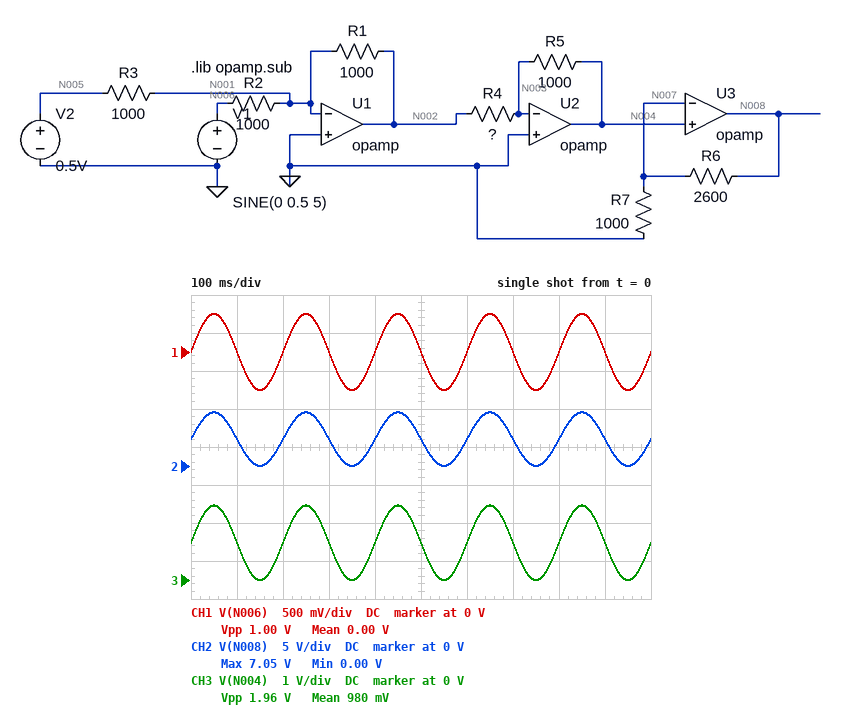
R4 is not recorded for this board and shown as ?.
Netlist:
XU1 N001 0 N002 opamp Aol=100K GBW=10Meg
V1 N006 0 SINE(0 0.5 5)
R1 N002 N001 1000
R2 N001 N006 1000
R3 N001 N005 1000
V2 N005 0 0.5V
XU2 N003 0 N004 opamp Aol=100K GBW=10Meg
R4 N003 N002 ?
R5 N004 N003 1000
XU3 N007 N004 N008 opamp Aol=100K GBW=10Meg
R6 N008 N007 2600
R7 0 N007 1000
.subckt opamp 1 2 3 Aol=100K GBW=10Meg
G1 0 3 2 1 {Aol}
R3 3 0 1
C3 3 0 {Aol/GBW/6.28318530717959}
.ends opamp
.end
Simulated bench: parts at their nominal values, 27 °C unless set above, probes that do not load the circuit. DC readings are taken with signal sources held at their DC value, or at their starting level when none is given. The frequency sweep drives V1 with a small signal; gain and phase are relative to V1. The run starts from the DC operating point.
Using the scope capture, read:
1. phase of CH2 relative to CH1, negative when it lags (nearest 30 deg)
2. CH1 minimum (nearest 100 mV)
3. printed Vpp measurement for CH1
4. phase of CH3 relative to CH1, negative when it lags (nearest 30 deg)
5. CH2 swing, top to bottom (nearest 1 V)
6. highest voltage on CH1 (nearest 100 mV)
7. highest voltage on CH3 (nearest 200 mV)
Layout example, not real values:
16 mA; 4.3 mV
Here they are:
0 deg; -500 mV; 1.00 V; 0 deg; 7 V; 500 mV; 2.0 V
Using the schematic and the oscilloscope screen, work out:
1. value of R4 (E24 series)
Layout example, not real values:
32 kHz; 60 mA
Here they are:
510 Ω
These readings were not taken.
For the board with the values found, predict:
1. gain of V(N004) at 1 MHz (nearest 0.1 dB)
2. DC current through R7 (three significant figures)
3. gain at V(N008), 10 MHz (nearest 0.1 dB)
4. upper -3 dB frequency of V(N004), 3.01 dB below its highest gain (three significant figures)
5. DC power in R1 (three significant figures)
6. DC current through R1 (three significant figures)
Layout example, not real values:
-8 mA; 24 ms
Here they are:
5.1 dB; 980 µA; -14.4 dB; 2.16 MHz; 250 µW; 500 µA
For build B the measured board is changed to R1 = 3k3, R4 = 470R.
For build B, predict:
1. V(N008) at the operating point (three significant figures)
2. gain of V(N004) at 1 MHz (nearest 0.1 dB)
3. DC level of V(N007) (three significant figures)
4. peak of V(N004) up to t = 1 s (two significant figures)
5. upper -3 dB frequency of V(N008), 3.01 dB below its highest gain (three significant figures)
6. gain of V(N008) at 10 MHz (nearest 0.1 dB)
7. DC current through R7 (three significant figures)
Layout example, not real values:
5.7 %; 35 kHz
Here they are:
12.6 V; 14.5 dB; 3.51 V; 7.0 V; 1.02 MHz; -11.4 dB; 3.51 mA
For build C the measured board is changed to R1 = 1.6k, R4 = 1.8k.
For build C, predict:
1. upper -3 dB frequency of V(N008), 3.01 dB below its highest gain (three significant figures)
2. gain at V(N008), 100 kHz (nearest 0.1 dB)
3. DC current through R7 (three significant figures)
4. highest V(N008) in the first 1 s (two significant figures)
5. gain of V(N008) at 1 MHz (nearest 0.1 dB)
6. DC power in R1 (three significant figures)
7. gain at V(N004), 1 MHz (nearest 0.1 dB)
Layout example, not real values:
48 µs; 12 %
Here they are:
1.57 MHz; 10.1 dB; 444 µA; 3.2 V; 8.8 dB; 400 µW; -1.8 dB
